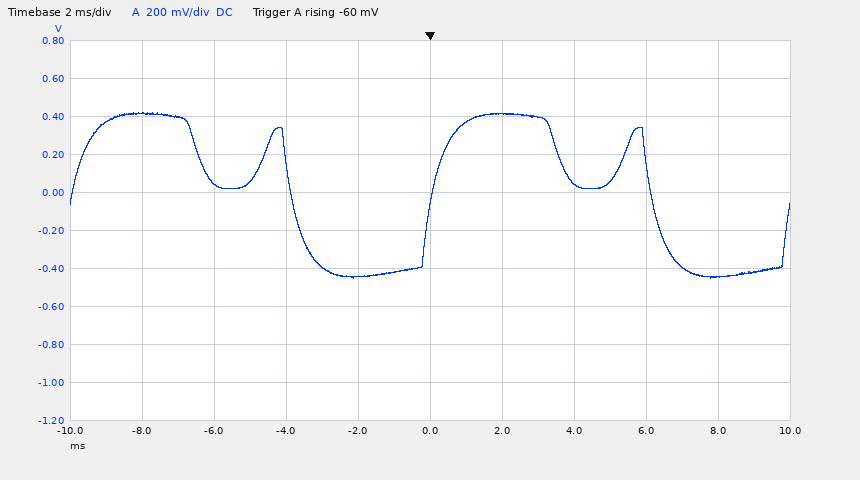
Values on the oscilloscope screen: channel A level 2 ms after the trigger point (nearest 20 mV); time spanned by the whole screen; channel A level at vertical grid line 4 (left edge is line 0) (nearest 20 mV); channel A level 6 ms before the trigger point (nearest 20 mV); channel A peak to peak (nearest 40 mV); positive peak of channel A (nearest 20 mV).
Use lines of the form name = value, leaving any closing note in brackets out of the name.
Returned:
channel A level 2 ms after the trigger point = 420 mV
time spanned by the whole screen = 20 ms
channel A level at vertical grid line 4 (left edge is line 0) = -440 mV
channel A level 6 ms before the trigger point = 40 mV
channel A peak to peak = 880 mV
positive peak of channel A = 420 mV
